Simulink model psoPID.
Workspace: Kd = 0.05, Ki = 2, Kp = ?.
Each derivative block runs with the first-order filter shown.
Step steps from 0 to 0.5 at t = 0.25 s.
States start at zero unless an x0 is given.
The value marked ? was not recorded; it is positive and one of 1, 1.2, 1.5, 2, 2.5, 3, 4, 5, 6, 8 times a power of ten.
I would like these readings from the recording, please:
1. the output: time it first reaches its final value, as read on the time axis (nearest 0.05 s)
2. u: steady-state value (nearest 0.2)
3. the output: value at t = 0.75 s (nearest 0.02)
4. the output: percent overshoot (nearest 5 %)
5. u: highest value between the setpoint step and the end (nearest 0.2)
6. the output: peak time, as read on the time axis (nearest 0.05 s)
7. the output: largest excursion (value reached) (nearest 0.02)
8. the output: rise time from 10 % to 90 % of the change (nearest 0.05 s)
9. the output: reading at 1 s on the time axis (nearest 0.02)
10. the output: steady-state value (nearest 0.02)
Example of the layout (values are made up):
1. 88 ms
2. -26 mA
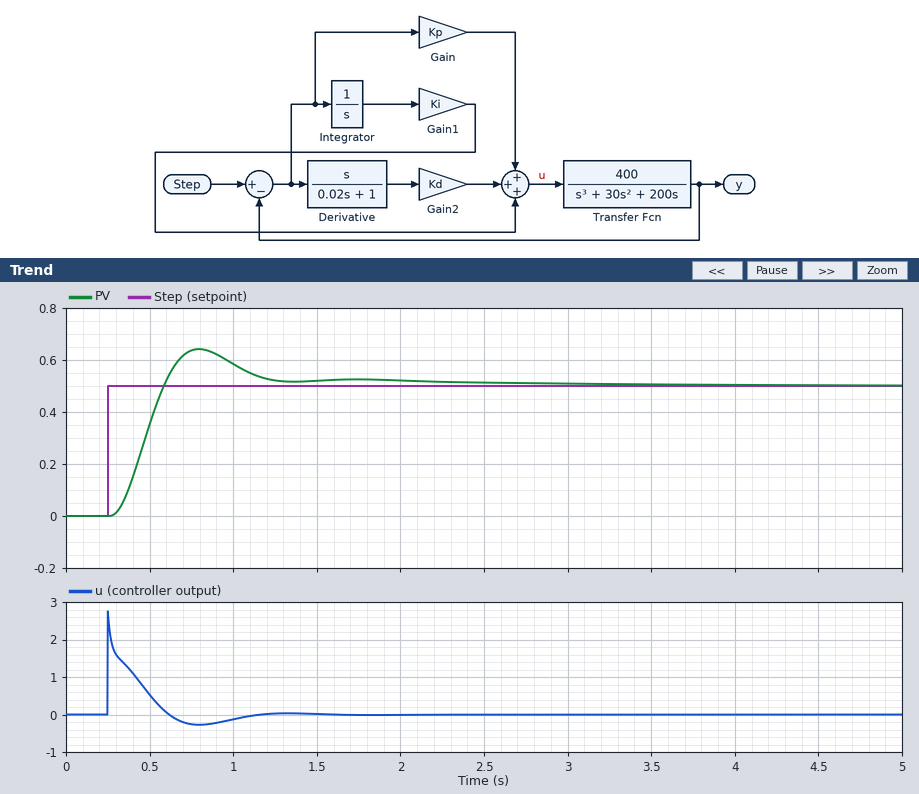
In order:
1. 0.60 s
2. 0.0
3. 0.64
4. 30 %
5. 2.8
6. 0.80 s
7. 0.64
8. 0.20 s
9. 0.58
10. 0.50
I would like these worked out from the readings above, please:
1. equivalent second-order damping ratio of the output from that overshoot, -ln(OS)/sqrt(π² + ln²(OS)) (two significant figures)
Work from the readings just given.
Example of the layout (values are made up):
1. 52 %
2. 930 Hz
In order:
1. 0.36
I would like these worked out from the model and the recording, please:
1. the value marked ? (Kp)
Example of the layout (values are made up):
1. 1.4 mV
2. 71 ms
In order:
1. 3
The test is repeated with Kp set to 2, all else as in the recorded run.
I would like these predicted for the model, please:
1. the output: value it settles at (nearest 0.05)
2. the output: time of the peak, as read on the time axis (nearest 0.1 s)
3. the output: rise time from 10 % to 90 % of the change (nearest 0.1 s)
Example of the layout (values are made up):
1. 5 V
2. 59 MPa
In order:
1. 0.50
2. 1.0 s
3. 0.3 s
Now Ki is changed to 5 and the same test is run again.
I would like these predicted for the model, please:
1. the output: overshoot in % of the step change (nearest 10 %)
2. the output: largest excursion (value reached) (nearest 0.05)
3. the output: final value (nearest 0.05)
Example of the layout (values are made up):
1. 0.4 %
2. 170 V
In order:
1. 50 %
2. 0.75
3. 0.50
